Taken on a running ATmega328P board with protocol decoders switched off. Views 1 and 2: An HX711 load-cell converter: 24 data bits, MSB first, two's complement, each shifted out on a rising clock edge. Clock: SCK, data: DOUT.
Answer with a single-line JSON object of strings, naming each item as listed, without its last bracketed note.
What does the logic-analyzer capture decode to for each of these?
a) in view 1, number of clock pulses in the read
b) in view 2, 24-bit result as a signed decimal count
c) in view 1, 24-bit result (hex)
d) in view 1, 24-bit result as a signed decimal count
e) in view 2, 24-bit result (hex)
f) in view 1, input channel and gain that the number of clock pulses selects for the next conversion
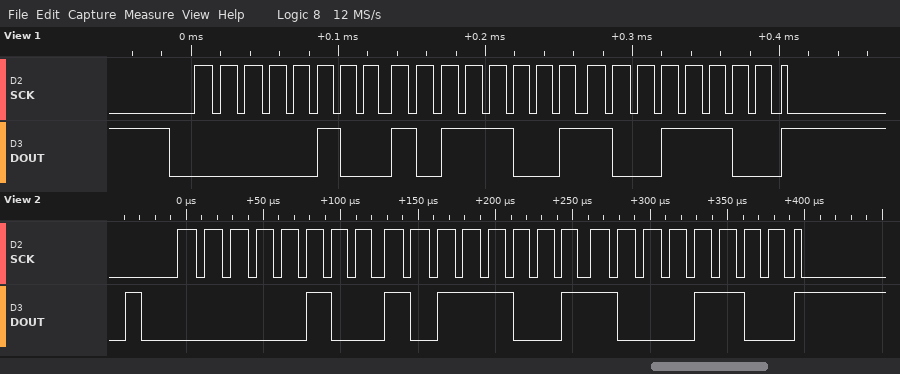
{"in view 1, number of clock pulses in the read": "25", "in view 2, 24-bit result as a signed decimal count": "309644", "in view 1, 24-bit result": "0x04B99C", "in view 1, 24-bit result as a signed decimal count": "309660", "in view 2, 24-bit result": "0x04B98C", "in view 1, input channel and gain that the number of clock pulses selects for the next conversion": "channel A, gain 128"}
